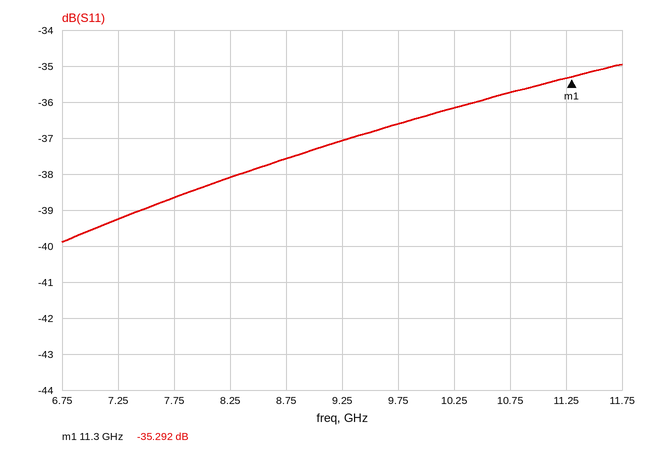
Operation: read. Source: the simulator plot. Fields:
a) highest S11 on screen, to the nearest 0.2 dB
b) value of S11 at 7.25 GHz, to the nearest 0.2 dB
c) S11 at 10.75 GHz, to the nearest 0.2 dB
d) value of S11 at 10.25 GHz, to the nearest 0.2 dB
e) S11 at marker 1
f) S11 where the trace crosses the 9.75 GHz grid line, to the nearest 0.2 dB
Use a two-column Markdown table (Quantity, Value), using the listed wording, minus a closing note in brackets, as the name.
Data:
| Quantity | Value |
|---|---|
| highest S11 on screen, to the nearest 0.2 dB | -35.0 dB |
| value of S11 at 7.25 GHz, to the nearest 0.2 dB | -39.2 dB |
| S11 at 10.75 GHz, to the nearest 0.2 dB | -35.8 dB |
| value of S11 at 10.25 GHz, to the nearest 0.2 dB | -36.2 dB |
| S11 at marker 1 | -35.292 dB |
| S11 where the trace crosses the 9.75 GHz grid line, to the nearest 0.2 dB | -36.6 dB |
